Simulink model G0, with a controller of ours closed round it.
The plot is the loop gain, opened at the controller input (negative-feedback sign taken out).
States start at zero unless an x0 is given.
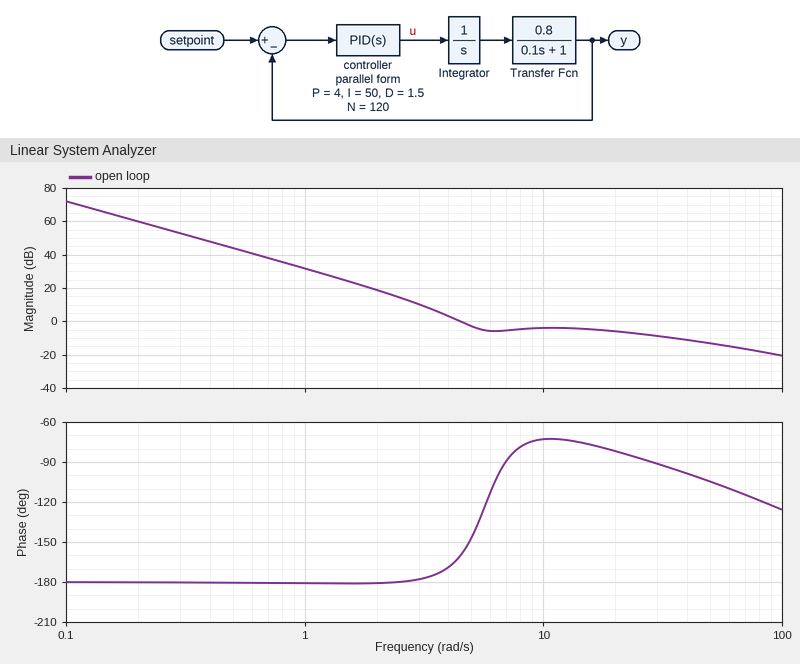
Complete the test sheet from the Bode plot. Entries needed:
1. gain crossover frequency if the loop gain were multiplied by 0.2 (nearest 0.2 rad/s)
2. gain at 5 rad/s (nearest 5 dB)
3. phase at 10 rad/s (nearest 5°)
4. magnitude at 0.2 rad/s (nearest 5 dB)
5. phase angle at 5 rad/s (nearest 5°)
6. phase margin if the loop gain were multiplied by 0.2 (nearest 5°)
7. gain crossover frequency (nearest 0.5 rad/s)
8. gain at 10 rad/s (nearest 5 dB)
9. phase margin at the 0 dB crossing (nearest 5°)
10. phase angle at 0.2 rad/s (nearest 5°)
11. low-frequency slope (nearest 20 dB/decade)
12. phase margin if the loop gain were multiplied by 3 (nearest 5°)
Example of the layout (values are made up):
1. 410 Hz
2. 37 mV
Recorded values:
1. 2.6 rad/s
2. -5 dB
3. -75°
4. 60 dB
5. -145°
6. 0°
7. 4.5 rad/s
8. -5 dB
9. 20°
10. -180°
11. -40 dB/decade
12. 85°
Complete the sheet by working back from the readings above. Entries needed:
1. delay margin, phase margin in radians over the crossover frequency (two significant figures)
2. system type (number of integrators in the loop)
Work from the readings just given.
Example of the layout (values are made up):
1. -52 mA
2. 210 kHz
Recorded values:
1. 0.078 s
2. 2
